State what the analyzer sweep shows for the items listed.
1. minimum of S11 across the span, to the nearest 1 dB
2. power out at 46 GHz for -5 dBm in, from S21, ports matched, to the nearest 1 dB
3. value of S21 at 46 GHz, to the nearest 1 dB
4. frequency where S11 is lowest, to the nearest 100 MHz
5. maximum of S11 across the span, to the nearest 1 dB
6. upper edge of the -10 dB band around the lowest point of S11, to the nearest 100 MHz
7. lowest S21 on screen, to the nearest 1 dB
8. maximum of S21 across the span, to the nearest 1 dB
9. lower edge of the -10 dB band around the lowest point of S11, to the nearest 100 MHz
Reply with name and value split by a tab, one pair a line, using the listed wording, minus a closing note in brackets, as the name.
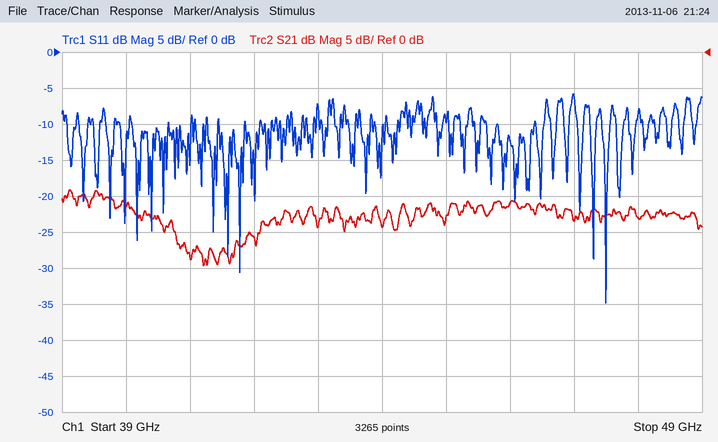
minimum of S11 across the span, to the nearest 1 dB	-35 dB
power out at 46 GHz for -5 dBm in, from S21, ports matched, to the nearest 1 dB	-26 dBm
value of S21 at 46 GHz, to the nearest 1 dB	-21 dB
frequency where S11 is lowest, to the nearest 100 MHz	47.5 GHz
maximum of S11 across the span, to the nearest 1 dB	-6 dB
upper edge of the -10 dB band around the lowest point of S11, to the nearest 100 MHz	47.6 GHz
lowest S21 on screen, to the nearest 1 dB	-30 dB
maximum of S21 across the span, to the nearest 1 dB	-19 dB
lower edge of the -10 dB band around the lowest point of S11, to the nearest 100 MHz	47.4 GHz
